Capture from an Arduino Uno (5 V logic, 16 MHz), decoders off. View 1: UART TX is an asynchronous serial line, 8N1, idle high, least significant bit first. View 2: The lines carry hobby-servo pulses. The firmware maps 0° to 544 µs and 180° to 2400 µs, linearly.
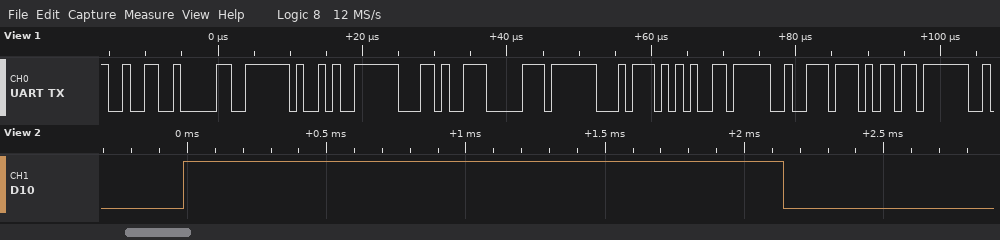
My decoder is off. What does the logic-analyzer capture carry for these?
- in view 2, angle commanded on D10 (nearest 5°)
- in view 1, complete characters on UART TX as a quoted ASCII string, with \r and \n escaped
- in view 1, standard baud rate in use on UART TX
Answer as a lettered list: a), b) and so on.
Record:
a) 155°
b) "20),pterm"
c) 1000000 baud
